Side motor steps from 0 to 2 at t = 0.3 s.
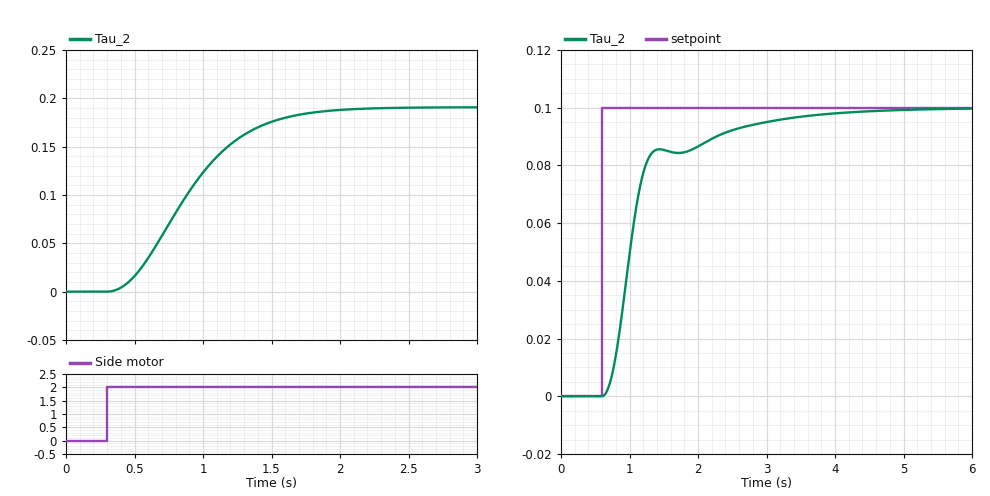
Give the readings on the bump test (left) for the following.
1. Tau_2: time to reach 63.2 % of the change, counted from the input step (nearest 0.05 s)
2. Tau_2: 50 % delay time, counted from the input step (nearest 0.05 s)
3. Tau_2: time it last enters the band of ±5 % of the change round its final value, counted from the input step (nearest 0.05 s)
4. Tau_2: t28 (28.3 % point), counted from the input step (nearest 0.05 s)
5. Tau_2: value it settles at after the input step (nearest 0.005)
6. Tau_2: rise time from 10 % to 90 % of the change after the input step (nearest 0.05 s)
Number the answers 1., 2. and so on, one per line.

1. 0.70 s
2. 0.55 s
3. 1.35 s
4. 0.40 s
5. 0.190
6. 0.90 s
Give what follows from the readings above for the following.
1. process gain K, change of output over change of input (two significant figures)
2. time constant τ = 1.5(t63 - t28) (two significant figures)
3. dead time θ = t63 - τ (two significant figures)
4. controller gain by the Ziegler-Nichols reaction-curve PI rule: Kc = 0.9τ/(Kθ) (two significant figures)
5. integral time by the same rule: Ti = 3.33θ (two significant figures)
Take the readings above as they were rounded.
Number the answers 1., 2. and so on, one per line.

1. 0.095
2. 0.45 s
3. 0.25 s
4. 17
5. 0.83 s
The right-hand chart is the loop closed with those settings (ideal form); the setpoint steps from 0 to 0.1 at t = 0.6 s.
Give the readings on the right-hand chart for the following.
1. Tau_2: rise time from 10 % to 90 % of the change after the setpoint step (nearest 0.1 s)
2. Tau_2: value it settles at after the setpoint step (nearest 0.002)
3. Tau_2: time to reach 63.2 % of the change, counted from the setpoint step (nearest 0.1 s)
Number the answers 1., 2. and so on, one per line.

1. 1.5 s
2. 0.100
3. 0.5 s
